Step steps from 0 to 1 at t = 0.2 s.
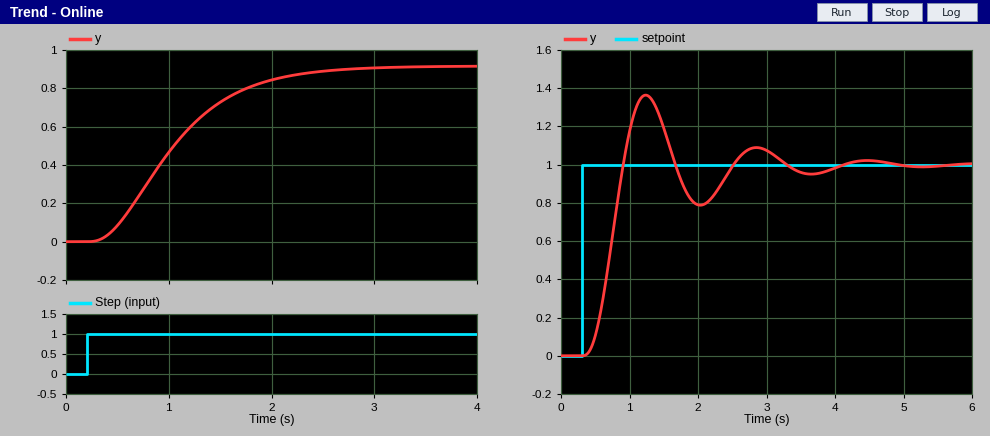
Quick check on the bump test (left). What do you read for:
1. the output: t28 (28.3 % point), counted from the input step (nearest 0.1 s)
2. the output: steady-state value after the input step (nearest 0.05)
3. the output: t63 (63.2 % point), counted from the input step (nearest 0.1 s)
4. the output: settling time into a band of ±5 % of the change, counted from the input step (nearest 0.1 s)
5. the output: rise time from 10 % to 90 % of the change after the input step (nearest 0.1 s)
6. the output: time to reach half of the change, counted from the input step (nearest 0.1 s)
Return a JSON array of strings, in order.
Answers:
["0.5 s", "0.90", "1.0 s", "2.0 s", "1.4 s", "0.8 s"]
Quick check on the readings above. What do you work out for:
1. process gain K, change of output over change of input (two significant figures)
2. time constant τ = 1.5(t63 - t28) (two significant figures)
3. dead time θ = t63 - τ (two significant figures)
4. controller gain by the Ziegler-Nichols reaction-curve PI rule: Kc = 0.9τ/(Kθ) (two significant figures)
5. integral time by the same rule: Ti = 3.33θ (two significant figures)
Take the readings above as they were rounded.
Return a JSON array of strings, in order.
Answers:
["0.90", "0.75 s", "0.25 s", "3.0", "0.83 s"]
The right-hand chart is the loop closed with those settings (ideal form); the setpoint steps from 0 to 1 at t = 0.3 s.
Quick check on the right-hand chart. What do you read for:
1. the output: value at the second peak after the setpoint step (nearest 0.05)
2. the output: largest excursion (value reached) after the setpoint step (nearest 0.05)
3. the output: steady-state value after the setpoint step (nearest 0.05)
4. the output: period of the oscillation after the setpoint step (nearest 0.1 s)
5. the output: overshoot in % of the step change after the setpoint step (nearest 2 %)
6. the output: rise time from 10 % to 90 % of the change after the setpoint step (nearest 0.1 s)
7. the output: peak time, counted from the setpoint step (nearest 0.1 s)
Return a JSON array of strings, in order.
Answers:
["1.10", "1.35", "1.00", "1.6 s", "36 %", "0.4 s", "0.9 s"]
